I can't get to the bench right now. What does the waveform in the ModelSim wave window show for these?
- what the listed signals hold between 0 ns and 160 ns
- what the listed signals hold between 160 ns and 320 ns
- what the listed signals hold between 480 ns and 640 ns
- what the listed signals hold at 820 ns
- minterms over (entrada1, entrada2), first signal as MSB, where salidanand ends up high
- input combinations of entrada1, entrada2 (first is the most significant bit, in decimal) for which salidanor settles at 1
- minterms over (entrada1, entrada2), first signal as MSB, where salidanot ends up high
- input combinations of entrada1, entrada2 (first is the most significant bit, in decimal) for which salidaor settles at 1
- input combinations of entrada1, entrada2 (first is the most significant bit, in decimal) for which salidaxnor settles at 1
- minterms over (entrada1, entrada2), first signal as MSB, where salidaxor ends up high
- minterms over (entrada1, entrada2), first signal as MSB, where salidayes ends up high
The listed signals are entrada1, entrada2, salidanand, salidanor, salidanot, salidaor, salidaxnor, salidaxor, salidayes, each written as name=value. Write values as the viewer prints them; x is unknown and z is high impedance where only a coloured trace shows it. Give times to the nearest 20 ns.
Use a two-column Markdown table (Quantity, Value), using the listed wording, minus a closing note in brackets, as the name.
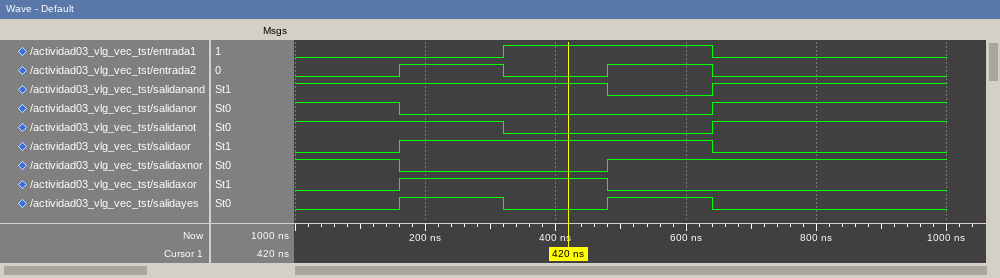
| Quantity | Value |
|---|---|
| what the listed signals hold between 0 ns and 160 ns | entrada1=0, entrada2=0, salidanand=1, salidanor=1, salidanot=1, salidaor=0, salidaxnor=1, salidaxor=0, salidayes=0 |
| what the listed signals hold between 160 ns and 320 ns | entrada1=0, entrada2=1, salidanand=1, salidanor=0, salidanot=1, salidaor=1, salidaxnor=0, salidaxor=1, salidayes=1 |
| what the listed signals hold between 480 ns and 640 ns | entrada1=1, entrada2=1, salidanand=0, salidanor=0, salidanot=0, salidaor=1, salidaxnor=1, salidaxor=0, salidayes=1 |
| what the listed signals hold at 820 ns | entrada1=0, entrada2=0, salidanand=1, salidanor=1, salidanot=1, salidaor=0, salidaxnor=1, salidaxor=0, salidayes=0 |
| minterms over (entrada1, entrada2), first signal as MSB, where salidanand ends up high | 0, 1, 2 |
| input combinations of entrada1, entrada2 (first is the most significant bit, in decimal) for which salidanor settles at 1 | 0 |
| minterms over (entrada1, entrada2), first signal as MSB, where salidanot ends up high | 0, 1 |
| input combinations of entrada1, entrada2 (first is the most significant bit, in decimal) for which salidaor settles at 1 | 1, 2, 3 |
| input combinations of entrada1, entrada2 (first is the most significant bit, in decimal) for which salidaxnor settles at 1 | 0, 3 |
| minterms over (entrada1, entrada2), first signal as MSB, where salidaxor ends up high | 1, 2 |
| minterms over (entrada1, entrada2), first signal as MSB, where salidayes ends up high | 1, 3 |
